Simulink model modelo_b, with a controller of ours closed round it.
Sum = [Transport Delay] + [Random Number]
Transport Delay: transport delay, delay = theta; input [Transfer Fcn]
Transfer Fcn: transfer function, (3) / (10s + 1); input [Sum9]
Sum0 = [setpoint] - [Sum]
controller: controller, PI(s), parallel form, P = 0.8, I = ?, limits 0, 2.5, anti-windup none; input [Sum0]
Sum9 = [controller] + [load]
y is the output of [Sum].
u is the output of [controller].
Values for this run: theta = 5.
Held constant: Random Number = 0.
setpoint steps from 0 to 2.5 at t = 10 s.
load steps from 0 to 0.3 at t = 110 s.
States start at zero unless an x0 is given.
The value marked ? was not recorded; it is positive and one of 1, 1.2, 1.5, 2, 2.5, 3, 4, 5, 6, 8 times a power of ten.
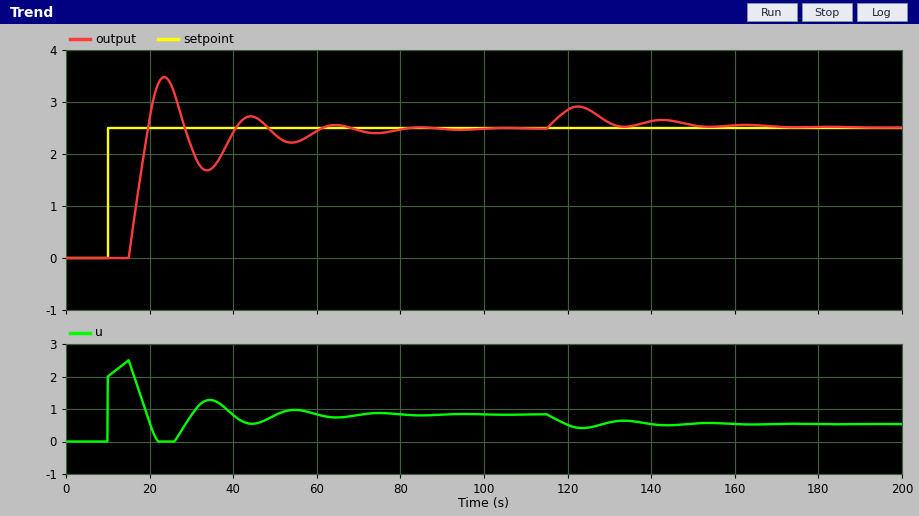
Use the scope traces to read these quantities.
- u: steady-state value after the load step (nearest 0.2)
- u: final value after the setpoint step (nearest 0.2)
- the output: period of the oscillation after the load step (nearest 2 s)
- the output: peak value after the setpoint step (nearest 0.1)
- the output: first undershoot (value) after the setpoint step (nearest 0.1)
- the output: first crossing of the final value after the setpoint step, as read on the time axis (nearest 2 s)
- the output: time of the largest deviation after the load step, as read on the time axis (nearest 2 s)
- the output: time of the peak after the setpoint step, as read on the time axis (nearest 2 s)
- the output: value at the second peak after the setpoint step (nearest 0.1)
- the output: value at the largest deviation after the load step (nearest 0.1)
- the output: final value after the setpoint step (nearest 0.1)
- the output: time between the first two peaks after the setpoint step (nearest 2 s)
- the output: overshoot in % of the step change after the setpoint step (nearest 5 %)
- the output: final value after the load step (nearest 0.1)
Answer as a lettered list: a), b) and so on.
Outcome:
a) 0.6
b) 0.8
c) 20 s
d) 3.5
e) 1.7
f) 20 s
g) 122 s
h) 24 s
i) 2.7
j) 2.9
k) 2.5
l) 20 s
m) 40 %
n) 2.5
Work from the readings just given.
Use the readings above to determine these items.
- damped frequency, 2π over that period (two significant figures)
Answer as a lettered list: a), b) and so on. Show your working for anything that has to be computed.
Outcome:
a) 2π / 20 = 0.31 rad/s
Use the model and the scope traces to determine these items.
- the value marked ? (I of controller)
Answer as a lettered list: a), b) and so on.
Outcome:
a) 0.04
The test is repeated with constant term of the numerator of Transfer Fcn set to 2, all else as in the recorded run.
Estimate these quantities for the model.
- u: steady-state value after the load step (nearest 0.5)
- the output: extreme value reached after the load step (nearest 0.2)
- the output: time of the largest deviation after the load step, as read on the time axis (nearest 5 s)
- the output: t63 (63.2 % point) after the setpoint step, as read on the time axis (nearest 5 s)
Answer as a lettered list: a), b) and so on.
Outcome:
a) 1.0
b) 2.8
c) 125 s
d) 20 s
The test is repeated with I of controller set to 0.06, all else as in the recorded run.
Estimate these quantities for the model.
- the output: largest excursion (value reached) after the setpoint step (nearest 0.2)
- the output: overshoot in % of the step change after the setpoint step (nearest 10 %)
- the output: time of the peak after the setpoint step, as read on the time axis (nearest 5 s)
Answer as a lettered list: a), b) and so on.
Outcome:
a) 3.8
b) 50 %
c) 25 s
